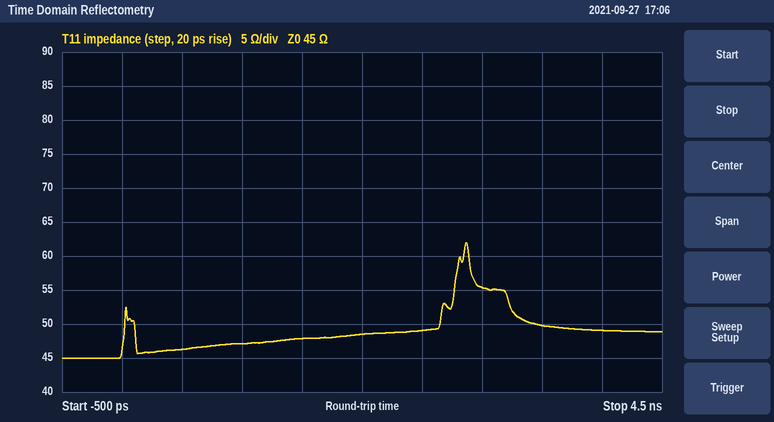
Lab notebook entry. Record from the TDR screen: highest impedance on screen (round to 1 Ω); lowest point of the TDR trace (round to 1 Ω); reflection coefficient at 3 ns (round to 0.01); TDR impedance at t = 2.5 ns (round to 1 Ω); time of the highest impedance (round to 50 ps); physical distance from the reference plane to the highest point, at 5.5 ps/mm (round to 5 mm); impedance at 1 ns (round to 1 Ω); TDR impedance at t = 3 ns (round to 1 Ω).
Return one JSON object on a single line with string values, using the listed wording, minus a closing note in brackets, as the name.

{"highest impedance on screen": "62 Ω", "lowest point of the TDR trace": "45 Ω", "reflection coefficient at 3 ns": "+0.10", "TDR impedance at t = 2.5 ns": "49 Ω", "time of the highest impedance": "2.85 ns", "physical distance from the reference plane to the highest point, at 5.5 ps/mm": "260 mm", "impedance at 1 ns": "47 Ω", "TDR impedance at t = 3 ns": "55 Ω"}
